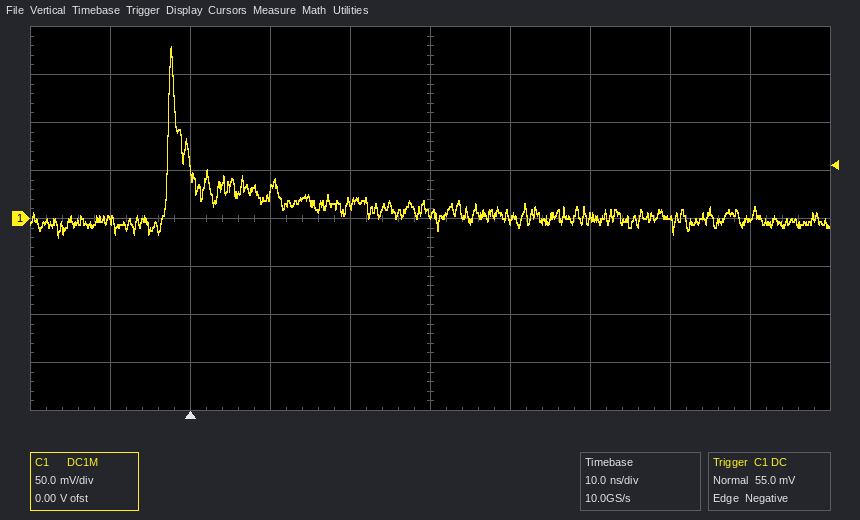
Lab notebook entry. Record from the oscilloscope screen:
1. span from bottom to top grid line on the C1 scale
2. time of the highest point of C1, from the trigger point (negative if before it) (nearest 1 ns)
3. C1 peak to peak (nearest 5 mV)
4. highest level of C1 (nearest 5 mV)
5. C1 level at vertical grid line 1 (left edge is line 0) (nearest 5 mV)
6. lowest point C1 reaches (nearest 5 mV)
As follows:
400 mV
-2 ns
200 mV
180 mV
0 mV
-20 mV
